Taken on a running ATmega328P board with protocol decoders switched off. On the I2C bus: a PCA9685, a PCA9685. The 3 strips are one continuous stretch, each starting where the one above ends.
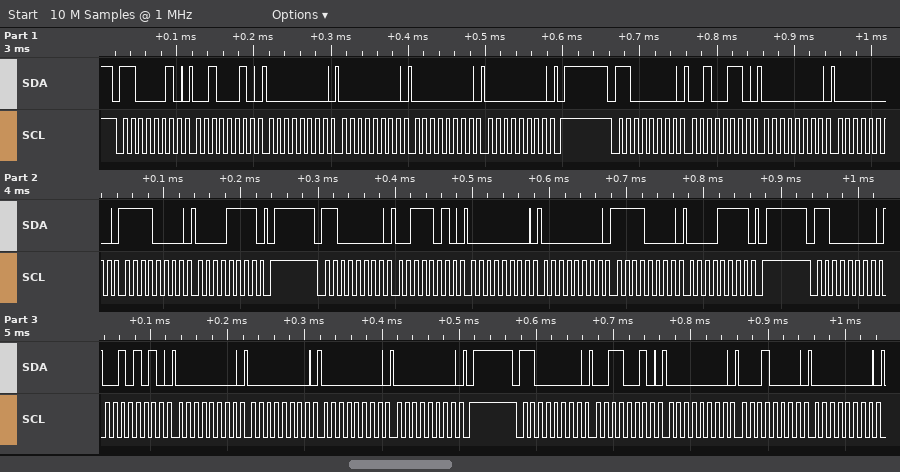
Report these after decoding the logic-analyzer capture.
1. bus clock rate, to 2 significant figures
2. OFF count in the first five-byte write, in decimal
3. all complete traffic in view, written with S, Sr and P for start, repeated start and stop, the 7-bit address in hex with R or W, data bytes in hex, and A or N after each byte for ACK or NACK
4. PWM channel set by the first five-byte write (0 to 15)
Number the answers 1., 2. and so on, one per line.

1. 100 kHz
2. 0
3. S 61W A 22 A 00 A 00 A 00 A 00 A P S 60W A 26 A 00 A 00 A F0 A 0F A P S 60W A 3A A 00 A 00 A F0 A 0F A P S 60W A 2A A 00 A 00 A 00 A 00 A P S 60W A 32 A 00 A 10 A 00 A
4. 7
